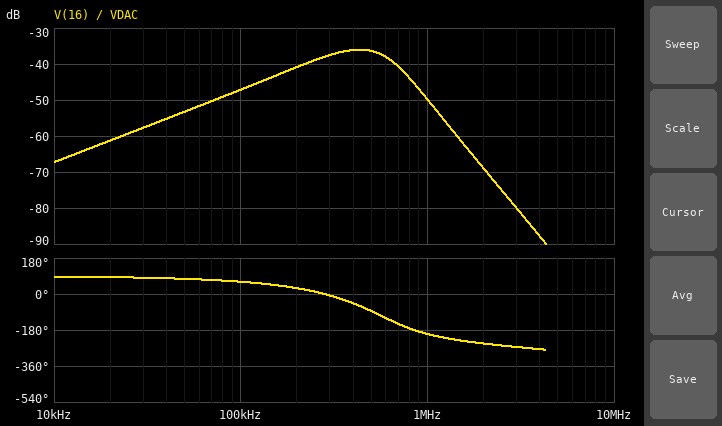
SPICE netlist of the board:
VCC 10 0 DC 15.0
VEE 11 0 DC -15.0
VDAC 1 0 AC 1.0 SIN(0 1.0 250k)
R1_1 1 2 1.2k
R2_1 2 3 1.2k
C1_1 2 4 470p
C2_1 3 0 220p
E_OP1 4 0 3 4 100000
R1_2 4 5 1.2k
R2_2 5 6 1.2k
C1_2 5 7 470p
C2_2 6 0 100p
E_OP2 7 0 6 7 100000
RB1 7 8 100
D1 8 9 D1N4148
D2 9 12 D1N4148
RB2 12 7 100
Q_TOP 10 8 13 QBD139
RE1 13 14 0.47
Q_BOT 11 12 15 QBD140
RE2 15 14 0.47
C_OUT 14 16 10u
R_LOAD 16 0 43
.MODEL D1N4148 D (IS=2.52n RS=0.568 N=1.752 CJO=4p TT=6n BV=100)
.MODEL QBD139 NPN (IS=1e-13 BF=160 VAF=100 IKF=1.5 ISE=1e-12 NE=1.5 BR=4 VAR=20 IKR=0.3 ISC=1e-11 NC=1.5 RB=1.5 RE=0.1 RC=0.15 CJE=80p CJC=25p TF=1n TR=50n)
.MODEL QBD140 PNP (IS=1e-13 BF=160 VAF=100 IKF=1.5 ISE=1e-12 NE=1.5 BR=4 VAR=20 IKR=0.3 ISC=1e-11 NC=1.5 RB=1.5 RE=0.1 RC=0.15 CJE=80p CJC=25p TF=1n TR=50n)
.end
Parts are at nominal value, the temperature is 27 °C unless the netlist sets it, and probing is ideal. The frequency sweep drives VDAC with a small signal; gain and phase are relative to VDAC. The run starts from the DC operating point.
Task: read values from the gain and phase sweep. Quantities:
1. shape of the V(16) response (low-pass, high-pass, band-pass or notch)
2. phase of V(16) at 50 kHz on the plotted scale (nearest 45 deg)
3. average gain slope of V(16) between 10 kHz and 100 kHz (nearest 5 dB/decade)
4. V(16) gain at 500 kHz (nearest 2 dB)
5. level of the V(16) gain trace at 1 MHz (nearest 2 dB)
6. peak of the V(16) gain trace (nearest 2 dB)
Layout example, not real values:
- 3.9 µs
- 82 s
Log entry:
- band-pass
- 90 deg
- 20 dB/decade
- -36 dB
- -50 dB
- -36 dB
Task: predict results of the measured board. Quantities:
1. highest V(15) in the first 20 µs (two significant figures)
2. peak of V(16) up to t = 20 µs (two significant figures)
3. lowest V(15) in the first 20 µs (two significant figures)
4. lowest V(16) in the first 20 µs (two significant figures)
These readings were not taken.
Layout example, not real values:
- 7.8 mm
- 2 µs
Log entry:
- 390 mV
- 390 mV
- -390 mV
- -390 mV
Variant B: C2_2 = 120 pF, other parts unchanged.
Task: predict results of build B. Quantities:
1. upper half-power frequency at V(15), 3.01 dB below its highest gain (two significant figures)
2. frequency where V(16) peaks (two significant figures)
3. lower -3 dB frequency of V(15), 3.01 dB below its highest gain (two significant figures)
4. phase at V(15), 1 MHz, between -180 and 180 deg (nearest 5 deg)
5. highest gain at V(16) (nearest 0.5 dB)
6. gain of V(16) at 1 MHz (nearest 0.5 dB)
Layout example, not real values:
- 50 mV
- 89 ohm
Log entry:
- 590 kHz
- 400 kHz
- 230 kHz
- 160 deg
- -36.5 dB
- -52.0 dB
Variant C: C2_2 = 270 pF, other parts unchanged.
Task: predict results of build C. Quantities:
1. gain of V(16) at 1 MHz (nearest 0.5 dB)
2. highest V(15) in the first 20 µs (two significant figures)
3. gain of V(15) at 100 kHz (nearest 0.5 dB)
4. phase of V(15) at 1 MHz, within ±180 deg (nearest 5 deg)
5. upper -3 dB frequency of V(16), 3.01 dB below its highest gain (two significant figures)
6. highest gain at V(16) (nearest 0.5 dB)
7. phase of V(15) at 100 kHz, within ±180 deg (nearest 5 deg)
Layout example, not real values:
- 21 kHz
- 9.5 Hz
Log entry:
- -60.0 dB
- 190 mV
- -47.5 dB
- 150 deg
- 460 kHz
- -40.5 dB
- 45 deg
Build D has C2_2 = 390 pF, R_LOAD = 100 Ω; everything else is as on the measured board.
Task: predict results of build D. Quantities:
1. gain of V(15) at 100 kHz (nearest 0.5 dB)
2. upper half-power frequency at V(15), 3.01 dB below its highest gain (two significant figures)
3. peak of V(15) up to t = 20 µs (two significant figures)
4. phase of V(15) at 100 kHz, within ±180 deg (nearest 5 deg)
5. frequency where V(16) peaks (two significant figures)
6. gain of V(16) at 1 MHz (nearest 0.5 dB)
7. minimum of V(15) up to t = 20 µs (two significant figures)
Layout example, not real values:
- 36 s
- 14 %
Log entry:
- -40.5 dB
- 430 kHz
- 80 mV
- 35 deg
- 260 kHz
- -56.5 dB
- -57 mV
